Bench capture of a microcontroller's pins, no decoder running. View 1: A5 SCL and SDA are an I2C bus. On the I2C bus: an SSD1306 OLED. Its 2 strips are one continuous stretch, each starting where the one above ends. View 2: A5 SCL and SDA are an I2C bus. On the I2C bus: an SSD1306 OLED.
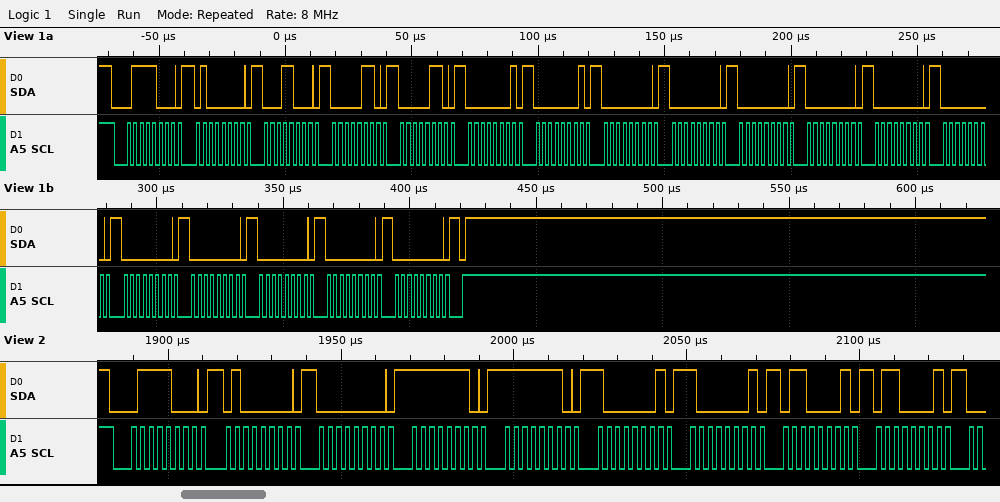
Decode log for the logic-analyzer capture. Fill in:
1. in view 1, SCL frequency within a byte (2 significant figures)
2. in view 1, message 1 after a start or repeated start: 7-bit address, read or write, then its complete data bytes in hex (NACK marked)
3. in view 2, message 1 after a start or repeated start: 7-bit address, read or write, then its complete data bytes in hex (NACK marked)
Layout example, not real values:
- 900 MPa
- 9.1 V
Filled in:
- 400 kHz
- 0x3C write: 40 18 06 06 01 01 00 00 00 00 00 00 00 00 00 00 00
- 0x3C write: 40 00 FE FE 81 81 61 61
